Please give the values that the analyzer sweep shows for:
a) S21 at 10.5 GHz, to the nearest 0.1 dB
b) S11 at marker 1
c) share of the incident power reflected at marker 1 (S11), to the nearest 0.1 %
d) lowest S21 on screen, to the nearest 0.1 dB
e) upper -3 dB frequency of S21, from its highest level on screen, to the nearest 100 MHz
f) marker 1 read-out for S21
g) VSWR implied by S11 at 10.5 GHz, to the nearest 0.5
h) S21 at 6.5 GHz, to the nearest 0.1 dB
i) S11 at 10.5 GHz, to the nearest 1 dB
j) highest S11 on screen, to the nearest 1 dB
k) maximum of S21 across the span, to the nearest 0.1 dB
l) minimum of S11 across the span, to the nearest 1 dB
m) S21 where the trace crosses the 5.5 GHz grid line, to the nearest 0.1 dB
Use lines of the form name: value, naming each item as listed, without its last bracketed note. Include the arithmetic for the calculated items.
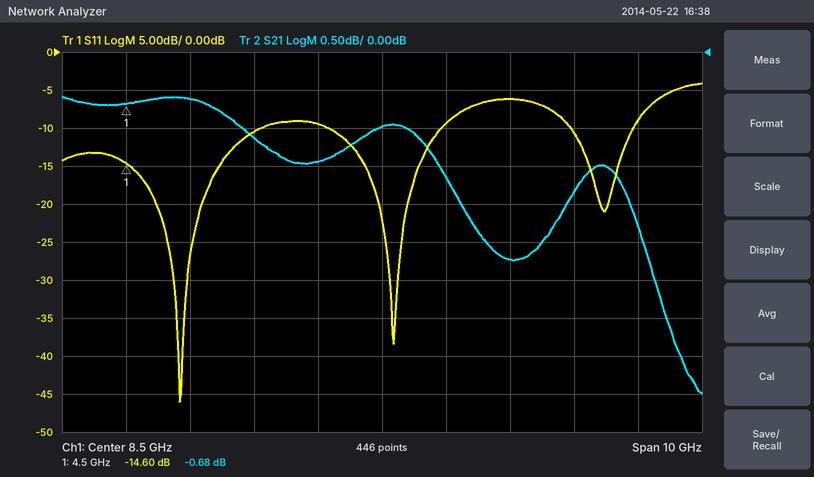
S21 at 10.5 GHz, to the nearest 0.1 dB: -2.7 dB
S11 at marker 1: -14.60 dB
share of the incident power reflected at marker 1 (S11), to the nearest 0.1 %: 10^(-14.6/10) ≈ 3.5 %
lowest S21 on screen, to the nearest 0.1 dB: -4.5 dB
upper -3 dB frequency of S21, from its highest level on screen, to the nearest 100 MHz: 13.0 GHz
marker 1 read-out for S21: -0.68 dB
VSWR implied by S11 at 10.5 GHz, to the nearest 0.5: |Γ| = 10^(-6/20) = 0.5012; VSWR = (1 + 0.5012)/(1 − 0.5012) ≈ 3.0
S21 at 6.5 GHz, to the nearest 0.1 dB: -1.1 dB
S11 at 10.5 GHz, to the nearest 1 dB: -6 dB
highest S11 on screen, to the nearest 1 dB: -4 dB
maximum of S21 across the span, to the nearest 0.1 dB: -0.6 dB
minimum of S11 across the span, to the nearest 1 dB: -46 dB
S21 where the trace crosses the 5.5 GHz grid line, to the nearest 0.1 dB: -0.6 dB
